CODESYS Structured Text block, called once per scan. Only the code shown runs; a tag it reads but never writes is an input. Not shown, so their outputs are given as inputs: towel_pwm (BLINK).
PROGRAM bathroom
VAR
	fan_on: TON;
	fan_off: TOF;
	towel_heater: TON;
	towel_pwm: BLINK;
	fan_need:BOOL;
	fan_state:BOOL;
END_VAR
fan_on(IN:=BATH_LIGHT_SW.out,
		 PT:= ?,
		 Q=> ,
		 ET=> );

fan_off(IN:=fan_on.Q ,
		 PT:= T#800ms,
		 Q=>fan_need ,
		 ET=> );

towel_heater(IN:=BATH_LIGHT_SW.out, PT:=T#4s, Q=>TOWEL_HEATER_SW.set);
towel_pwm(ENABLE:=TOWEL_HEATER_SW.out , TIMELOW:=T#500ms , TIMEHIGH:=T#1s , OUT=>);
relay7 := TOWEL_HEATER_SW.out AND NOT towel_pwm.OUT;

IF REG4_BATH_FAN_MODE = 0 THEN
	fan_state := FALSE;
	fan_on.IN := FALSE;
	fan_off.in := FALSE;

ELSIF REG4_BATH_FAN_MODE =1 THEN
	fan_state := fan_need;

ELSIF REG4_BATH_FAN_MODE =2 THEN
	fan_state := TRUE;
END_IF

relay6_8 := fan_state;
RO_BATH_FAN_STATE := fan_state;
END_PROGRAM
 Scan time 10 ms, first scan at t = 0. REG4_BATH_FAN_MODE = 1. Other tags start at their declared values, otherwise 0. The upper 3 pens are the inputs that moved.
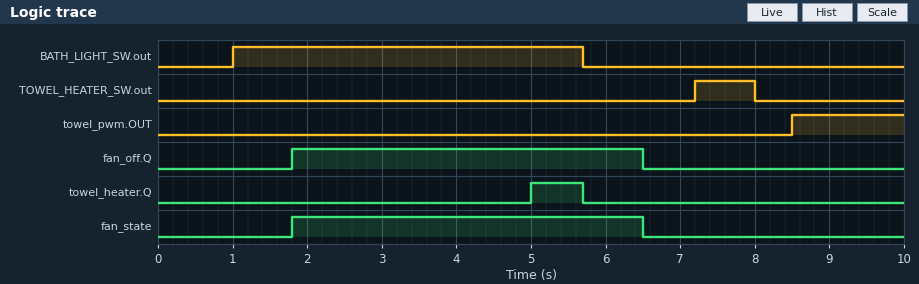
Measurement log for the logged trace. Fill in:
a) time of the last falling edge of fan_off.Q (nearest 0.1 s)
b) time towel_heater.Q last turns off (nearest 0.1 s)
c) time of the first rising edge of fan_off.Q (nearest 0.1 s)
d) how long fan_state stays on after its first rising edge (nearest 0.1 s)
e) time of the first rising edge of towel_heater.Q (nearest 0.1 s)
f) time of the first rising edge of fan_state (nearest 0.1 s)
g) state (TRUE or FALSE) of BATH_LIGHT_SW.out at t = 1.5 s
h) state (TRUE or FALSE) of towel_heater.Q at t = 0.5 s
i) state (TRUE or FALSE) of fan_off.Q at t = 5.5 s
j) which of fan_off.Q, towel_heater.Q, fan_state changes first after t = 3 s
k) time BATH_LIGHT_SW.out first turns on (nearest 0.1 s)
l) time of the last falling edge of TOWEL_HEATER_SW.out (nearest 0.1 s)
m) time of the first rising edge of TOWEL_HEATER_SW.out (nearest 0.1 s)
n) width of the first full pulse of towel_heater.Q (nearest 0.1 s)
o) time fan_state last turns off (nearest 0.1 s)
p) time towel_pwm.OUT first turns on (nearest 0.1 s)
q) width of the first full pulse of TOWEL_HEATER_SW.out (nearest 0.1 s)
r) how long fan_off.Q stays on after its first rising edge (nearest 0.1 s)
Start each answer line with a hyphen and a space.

- 6.5 s
- 5.7 s
- 1.8 s
- 4.7 s
- 5.0 s
- 1.8 s
- TRUE
- FALSE
- TRUE
- towel_heater.Q
- 1.0 s
- 8.0 s
- 7.2 s
- 0.7 s
- 6.5 s
- 8.5 s
- 0.8 s
- 4.7 s
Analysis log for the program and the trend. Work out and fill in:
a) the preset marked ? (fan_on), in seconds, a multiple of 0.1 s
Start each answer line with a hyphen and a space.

- 0.8 s
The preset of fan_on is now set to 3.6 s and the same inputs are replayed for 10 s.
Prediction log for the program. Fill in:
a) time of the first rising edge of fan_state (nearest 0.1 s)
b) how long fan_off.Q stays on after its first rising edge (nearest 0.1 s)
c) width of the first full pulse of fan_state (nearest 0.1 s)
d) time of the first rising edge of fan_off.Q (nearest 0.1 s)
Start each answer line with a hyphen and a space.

- 4.6 s
- 1.9 s
- 1.9 s
- 4.6 s
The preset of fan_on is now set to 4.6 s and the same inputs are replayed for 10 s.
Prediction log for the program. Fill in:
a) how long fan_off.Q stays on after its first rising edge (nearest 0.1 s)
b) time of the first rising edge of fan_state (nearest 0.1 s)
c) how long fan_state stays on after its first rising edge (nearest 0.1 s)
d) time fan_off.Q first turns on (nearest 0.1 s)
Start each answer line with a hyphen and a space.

- 0.9 s
- 5.6 s
- 0.9 s
- 5.6 s
